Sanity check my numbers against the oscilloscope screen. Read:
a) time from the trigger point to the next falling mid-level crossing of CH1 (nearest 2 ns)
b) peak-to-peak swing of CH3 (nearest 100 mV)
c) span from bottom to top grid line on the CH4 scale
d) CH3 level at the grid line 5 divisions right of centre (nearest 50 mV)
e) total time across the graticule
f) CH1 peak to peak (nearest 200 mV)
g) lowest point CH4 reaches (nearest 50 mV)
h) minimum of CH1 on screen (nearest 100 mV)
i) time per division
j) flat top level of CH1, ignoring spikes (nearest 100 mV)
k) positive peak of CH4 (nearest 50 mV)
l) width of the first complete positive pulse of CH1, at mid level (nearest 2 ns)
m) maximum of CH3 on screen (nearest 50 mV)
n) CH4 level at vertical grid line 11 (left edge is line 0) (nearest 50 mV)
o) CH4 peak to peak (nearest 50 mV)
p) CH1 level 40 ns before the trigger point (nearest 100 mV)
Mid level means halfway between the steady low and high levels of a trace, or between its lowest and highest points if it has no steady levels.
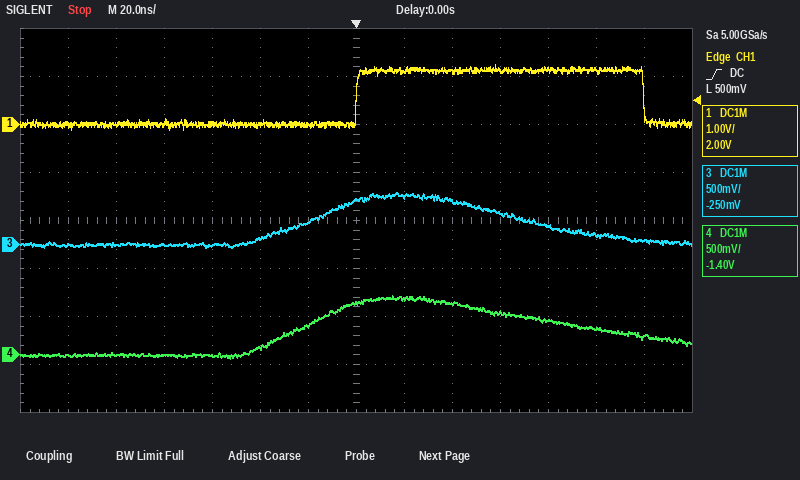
120 ns
600 mV
4 V
100 mV
280 ns
1.4 V
-50 mV
-100 mV
20 ns
1.1 V
600 mV
120 ns
550 mV
350 mV
650 mV
0.0 V
